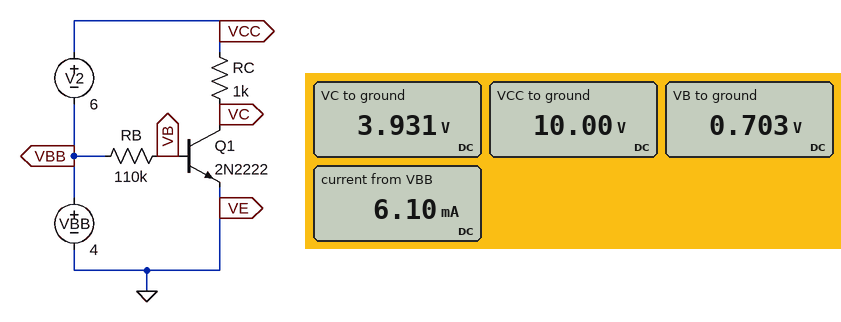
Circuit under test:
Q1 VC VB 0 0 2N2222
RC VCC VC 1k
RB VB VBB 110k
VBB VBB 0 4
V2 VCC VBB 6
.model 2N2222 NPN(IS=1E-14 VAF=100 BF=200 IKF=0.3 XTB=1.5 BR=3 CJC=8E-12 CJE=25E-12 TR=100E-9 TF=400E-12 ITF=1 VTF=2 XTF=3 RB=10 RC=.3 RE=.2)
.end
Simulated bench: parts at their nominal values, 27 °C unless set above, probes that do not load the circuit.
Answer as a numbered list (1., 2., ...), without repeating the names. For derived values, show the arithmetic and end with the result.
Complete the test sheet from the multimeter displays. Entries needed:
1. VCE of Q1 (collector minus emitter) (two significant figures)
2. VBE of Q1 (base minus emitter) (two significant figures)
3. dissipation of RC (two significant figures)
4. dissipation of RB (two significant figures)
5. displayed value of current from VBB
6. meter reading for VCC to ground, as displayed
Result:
1. 3.931 V = 3.9 V
2. 703 mV = 700 mV
3. (10 V - 3.931 V)^2 / 1 kΩ = 37 mW
4. (4 V - 703 mV)^2 / 110 kΩ = 99 µW
5. 6.10 mA
6. 10.00 V
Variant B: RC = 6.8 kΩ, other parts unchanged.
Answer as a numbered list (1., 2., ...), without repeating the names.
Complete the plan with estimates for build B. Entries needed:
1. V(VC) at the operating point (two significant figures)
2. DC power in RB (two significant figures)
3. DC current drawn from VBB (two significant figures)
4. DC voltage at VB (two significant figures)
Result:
1. 82 mV
2. 100 µW
3. 1.5 mA
4. 670 mV
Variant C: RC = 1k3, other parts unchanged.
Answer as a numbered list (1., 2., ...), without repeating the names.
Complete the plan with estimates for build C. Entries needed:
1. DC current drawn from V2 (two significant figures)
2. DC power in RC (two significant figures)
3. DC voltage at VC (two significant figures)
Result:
1. 6.0 mA
2. 46 mW
3. 2.2 V
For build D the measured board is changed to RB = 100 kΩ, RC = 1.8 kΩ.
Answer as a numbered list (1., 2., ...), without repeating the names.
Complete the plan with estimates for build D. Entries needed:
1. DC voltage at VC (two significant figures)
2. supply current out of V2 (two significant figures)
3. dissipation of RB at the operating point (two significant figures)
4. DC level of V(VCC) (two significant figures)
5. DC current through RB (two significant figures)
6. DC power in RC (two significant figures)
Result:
1. 160 mV
2. 5.5 mA
3. 110 µW
4. 10 V
5. 33 µA
6. 54 mW
